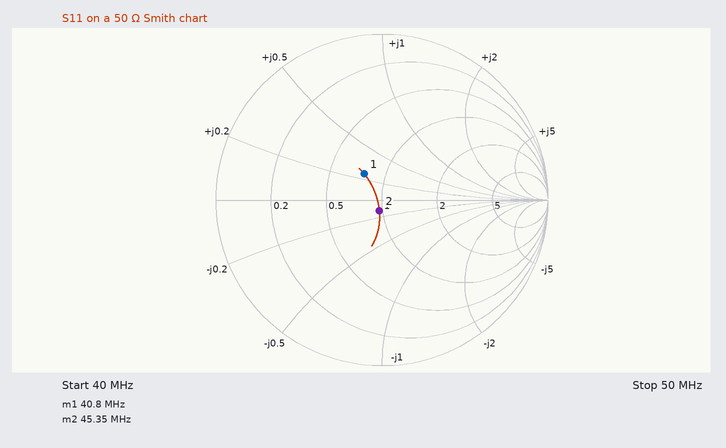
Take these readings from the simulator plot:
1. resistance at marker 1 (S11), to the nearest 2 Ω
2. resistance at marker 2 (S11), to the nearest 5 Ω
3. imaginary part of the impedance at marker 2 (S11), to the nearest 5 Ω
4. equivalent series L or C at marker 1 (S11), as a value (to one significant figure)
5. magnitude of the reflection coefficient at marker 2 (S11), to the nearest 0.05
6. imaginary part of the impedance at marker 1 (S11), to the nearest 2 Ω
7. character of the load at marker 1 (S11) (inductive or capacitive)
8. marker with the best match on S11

38 Ω
50 Ω
-5 Ω
50 nH
0.05
+12 Ω
inductive
marker 2
